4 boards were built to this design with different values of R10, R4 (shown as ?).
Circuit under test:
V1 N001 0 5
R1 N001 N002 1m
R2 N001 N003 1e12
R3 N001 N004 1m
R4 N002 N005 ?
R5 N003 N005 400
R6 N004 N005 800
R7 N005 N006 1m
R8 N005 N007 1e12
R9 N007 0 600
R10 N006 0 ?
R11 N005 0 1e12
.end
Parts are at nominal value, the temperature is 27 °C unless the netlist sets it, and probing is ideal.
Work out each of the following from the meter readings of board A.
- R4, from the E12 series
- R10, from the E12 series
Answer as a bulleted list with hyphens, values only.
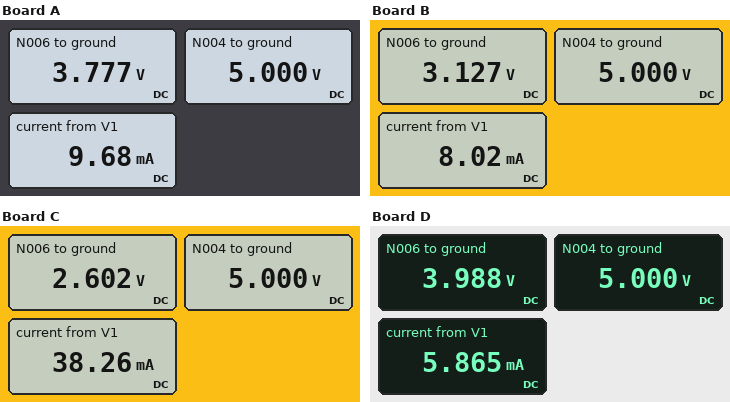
- 150 Ω
- 390 Ω
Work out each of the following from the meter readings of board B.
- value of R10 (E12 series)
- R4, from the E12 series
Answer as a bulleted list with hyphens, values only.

- 390 Ω
- 330 Ω
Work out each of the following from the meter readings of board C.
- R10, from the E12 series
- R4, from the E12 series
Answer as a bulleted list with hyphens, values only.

- 68 Ω
- 68 Ω
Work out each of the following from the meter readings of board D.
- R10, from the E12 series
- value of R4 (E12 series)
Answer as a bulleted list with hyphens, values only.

- 680 Ω
- 220 Ω
